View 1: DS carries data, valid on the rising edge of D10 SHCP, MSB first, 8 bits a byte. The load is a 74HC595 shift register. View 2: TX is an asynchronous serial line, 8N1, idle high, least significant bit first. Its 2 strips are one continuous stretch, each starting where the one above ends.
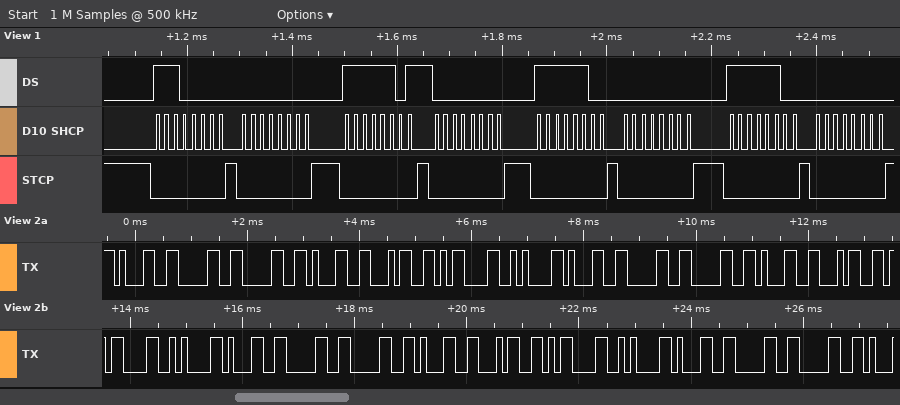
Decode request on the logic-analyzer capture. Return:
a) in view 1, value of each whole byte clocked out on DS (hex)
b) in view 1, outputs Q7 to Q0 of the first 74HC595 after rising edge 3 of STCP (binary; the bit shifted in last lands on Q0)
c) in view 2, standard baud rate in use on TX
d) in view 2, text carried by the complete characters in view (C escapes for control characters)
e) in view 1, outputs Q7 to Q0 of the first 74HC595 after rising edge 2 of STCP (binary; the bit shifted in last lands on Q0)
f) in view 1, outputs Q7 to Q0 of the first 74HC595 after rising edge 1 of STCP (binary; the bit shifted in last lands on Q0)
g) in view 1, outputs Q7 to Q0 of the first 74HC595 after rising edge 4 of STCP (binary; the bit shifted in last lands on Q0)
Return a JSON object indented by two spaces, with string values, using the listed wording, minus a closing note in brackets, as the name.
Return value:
{
  "in view 1, value of each whole byte clocked out on DS": "E0 00 FD 00 FC 00 FC 00",
  "in view 1, outputs Q7 to Q0 of the first 74HC595 after rising edge 3 of STCP": "11111101",
  "in view 2, standard baud rate in use on TX": "9600 baud",
  "in view 2, text carried by the complete characters in view": "\"10014\\r\\n10014\\r\\n10014\\r\\n100\"",
  "in view 1, outputs Q7 to Q0 of the first 74HC595 after rising edge 2 of STCP": "00000000",
  "in view 1, outputs Q7 to Q0 of the first 74HC595 after rising edge 1 of STCP": "11100000",
  "in view 1, outputs Q7 to Q0 of the first 74HC595 after rising edge 4 of STCP": "00000000"
}
